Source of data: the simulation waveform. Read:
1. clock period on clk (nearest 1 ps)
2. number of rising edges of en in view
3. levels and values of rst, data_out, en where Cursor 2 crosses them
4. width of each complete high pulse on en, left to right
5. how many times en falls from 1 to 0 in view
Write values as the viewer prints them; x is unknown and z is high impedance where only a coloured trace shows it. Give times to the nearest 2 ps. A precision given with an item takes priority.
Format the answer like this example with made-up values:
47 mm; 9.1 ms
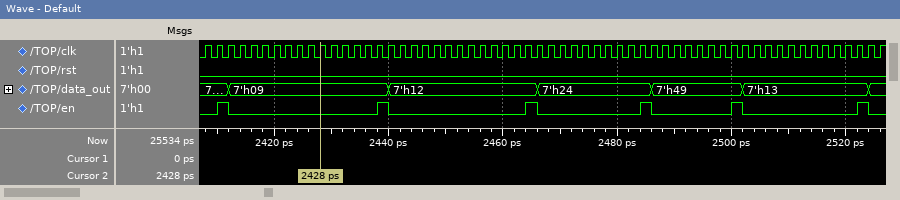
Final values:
2 ps; 6; rst=0, data_out=7'h09, en=0; 2 ps, 2 ps, 2 ps, 2 ps, 2 ps, 2 ps; 6
